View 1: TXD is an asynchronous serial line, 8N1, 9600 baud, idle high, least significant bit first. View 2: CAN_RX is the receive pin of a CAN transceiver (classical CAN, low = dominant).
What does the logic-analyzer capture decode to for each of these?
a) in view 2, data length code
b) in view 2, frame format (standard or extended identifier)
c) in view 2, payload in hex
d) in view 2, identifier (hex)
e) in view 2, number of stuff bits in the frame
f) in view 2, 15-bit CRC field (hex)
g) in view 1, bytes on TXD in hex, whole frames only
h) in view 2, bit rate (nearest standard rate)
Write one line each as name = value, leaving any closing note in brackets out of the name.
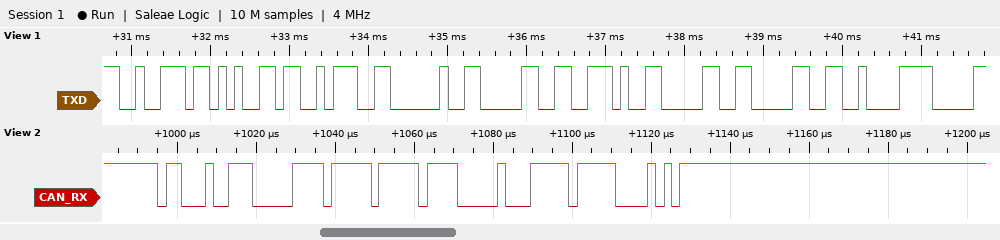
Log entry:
in view 2, data length code = 3
in view 2, frame format = standard
in view 2, payload in hex = BF FF 00
in view 2, identifier = 0x627
in view 2, number of stuff bits in the frame = 6
in view 2, 15-bit CRC field = 0x7FE2
in view 1, bytes on TXD in hex, whole frames only = 72 65 3A 20 30 2E 30 30 C2
in view 2, bit rate = 500 kbit/s
